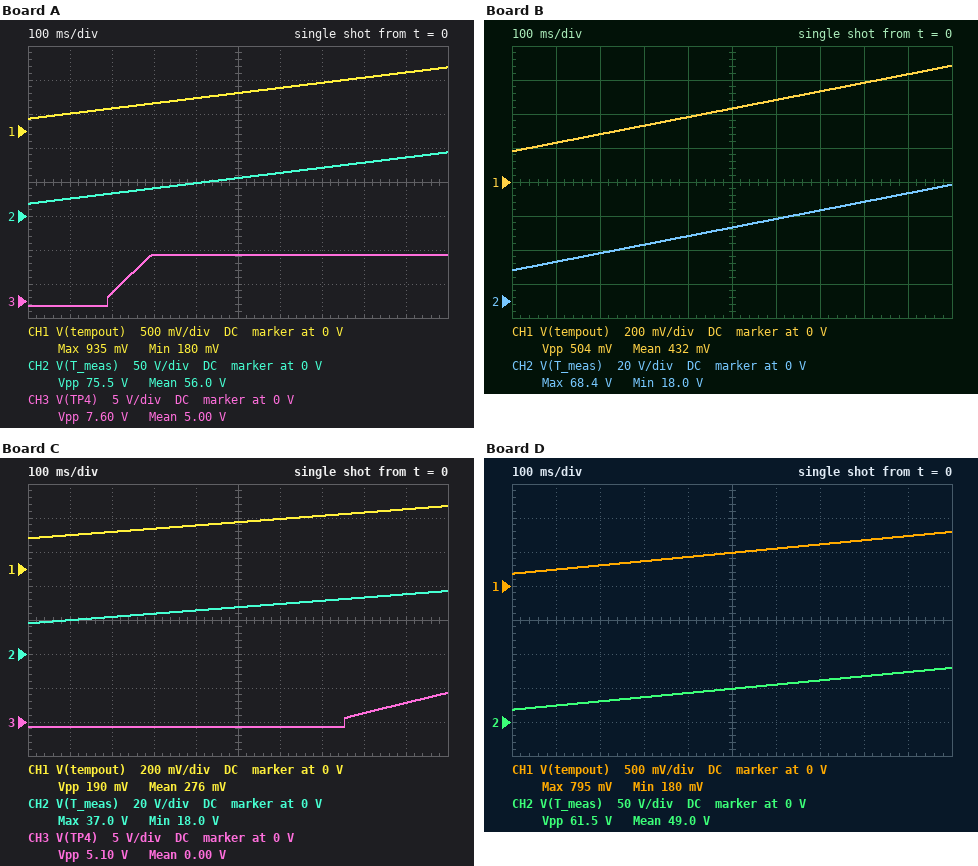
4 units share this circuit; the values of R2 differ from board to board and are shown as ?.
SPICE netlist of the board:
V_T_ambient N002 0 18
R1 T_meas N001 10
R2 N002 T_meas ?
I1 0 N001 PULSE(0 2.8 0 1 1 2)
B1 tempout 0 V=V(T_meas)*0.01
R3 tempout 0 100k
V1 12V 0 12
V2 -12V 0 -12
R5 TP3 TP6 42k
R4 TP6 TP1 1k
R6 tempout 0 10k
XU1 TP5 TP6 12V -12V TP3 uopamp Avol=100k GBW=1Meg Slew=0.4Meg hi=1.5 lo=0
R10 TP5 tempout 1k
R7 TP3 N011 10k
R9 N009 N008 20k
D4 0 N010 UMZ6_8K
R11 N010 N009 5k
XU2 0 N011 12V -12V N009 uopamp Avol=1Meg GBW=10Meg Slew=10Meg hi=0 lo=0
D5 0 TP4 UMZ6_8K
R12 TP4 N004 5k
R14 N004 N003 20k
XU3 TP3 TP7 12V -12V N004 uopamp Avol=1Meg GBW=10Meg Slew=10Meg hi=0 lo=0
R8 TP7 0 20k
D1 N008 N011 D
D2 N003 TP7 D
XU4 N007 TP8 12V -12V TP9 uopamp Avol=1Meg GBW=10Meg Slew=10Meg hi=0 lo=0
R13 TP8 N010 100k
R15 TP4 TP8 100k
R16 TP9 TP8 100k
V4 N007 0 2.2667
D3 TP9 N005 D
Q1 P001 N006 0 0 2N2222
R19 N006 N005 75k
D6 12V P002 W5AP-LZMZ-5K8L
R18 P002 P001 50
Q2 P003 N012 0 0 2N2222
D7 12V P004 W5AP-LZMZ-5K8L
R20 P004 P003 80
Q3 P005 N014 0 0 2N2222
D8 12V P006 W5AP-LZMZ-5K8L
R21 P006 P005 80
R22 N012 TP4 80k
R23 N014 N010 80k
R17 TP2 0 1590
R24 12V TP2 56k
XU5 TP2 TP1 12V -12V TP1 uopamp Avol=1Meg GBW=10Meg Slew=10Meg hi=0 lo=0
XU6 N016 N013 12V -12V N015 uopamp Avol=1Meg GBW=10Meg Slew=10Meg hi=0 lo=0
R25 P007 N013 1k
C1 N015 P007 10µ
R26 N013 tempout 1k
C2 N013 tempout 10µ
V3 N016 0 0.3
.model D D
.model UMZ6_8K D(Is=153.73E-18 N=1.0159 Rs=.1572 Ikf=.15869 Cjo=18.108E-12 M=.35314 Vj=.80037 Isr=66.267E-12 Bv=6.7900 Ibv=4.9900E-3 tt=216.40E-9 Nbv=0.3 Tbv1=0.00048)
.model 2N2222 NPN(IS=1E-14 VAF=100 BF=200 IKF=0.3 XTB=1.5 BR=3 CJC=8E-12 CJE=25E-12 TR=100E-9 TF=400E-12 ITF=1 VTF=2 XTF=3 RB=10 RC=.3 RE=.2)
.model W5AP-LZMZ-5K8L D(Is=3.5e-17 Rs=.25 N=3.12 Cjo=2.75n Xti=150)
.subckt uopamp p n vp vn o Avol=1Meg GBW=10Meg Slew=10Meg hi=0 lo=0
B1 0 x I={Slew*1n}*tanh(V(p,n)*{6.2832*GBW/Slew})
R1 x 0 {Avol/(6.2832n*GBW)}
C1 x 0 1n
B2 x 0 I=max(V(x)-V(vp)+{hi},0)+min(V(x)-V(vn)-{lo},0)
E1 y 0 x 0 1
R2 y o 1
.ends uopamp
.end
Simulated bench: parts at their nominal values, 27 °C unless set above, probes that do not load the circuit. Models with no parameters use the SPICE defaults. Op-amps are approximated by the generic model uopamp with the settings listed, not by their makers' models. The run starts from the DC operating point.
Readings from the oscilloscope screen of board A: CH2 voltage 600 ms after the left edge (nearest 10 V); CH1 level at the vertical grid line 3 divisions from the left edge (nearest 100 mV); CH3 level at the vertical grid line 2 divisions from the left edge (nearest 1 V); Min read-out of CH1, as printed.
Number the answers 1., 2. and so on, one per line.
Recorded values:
1. 60 V
2. 400 mV
3. 1 V
4. 180 mV
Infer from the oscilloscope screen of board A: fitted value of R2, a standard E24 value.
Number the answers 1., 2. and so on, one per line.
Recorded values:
1. 27 Ω
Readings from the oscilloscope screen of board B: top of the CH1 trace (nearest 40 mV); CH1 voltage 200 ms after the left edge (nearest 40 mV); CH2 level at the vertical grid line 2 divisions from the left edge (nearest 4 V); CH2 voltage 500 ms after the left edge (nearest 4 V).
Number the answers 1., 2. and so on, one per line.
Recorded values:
1. 680 mV
2. 280 mV
3. 28 V
4. 44 V
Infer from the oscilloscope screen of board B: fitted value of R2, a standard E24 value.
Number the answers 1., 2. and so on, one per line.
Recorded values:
1. 18 Ω
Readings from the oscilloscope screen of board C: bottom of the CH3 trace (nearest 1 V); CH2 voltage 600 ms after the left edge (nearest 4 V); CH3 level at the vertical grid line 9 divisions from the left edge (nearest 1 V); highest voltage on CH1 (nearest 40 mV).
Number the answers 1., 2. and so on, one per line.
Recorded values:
1. -1 V
2. 28 V
3. 3 V
4. 360 mV
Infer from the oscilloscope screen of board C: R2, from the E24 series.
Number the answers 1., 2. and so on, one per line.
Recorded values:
1. 6.8 Ω
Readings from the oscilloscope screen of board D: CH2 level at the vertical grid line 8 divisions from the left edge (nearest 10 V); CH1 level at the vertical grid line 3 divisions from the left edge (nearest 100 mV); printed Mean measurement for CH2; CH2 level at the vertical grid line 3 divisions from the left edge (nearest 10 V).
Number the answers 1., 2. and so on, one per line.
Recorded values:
1. 70 V
2. 400 mV
3. 49.0 V
4. 40 V
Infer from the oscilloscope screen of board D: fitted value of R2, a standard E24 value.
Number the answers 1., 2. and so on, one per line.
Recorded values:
1. 22 Ω
